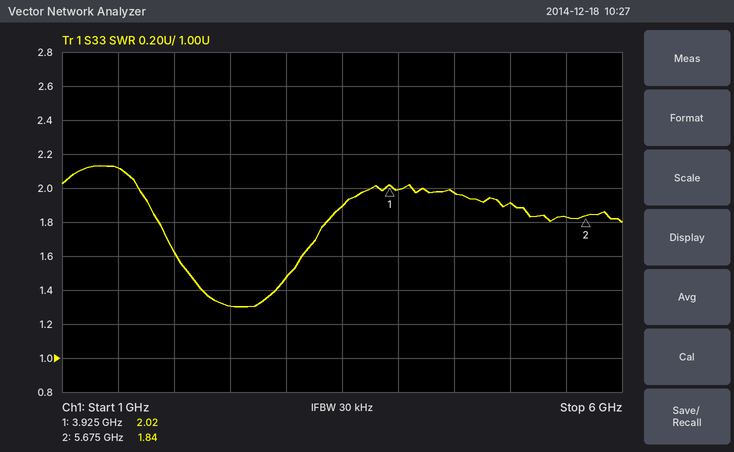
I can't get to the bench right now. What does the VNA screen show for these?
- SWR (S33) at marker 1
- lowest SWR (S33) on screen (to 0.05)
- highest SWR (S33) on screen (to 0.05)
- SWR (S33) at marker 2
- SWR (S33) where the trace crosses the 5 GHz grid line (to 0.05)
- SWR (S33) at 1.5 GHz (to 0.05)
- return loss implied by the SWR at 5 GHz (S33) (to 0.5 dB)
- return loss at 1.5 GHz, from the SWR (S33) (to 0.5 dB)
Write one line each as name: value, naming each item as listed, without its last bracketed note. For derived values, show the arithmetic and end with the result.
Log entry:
SWR (S33) at marker 1: 2.02
lowest SWR (S33) on screen: 1.30
highest SWR (S33) on screen: 2.15
SWR (S33) at marker 2: 1.84
SWR (S33) where the trace crosses the 5 GHz grid line: 1.90
SWR (S33) at 1.5 GHz: 2.10
return loss implied by the SWR at 5 GHz (S33): −20 log10((1.9 − 1)/(1.9 + 1)) ≈ 10.2 dB, so 10.0 dB to the nearest 0.5 dB
return loss at 1.5 GHz, from the SWR (S33): −20 log10((2.1 − 1)/(2.1 + 1)) ≈ 9.0 dB
